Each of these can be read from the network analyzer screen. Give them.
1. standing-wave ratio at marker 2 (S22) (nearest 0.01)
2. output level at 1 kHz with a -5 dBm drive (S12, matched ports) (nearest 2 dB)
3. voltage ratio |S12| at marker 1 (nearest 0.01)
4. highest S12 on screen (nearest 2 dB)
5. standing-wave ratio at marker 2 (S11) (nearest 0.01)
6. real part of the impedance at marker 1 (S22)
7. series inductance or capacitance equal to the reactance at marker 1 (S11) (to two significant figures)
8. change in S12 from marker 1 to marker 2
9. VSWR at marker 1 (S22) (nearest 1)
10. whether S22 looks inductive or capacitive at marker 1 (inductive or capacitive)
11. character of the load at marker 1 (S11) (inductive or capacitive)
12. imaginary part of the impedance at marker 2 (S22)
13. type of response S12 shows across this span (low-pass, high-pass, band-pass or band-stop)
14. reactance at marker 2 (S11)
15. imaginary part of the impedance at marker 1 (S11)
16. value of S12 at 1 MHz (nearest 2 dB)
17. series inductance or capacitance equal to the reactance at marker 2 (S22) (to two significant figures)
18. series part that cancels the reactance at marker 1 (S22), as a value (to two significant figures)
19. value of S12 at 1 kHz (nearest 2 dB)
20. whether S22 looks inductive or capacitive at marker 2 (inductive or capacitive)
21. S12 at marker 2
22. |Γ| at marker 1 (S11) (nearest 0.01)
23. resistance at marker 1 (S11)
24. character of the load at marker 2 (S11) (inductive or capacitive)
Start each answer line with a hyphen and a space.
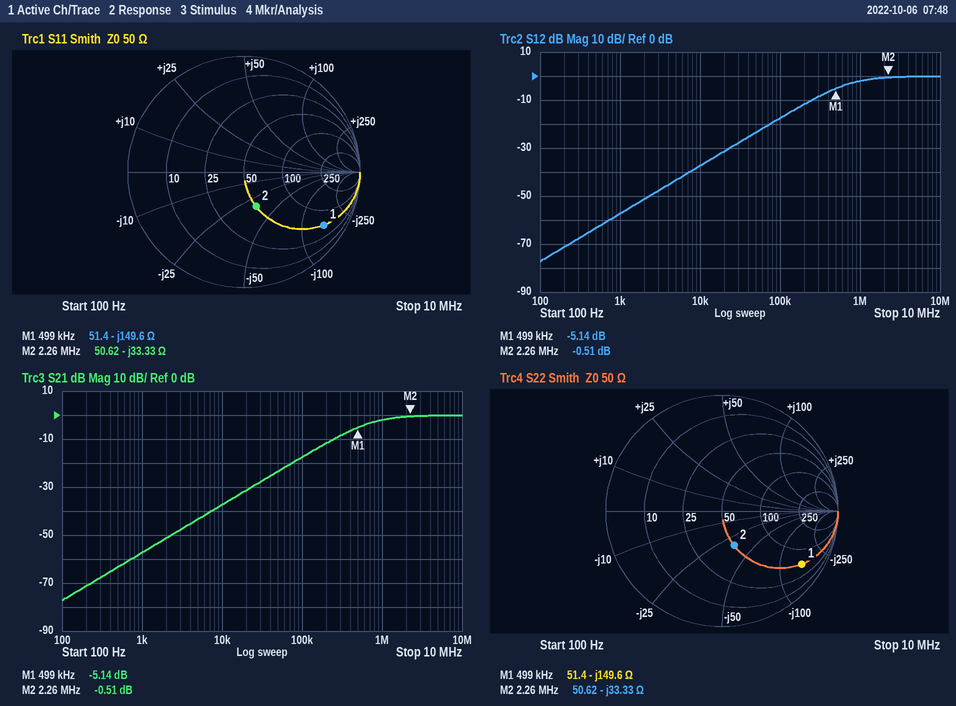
- 1.92
- -62 dBm
- 0.55
- 0 dB
- 1.92
- 51.4 Ω
- 2.1 nF
- 4.63 dB
- 11
- capacitive
- capacitive
- -33.33 Ω
- high-pass
- -33.33 Ω
- -149.6 Ω
- -2 dB
- 2.1 nF
- 48 µH
- -58 dB
- capacitive
- -0.51 dB
- 0.83
- 51.4 Ω
- capacitive
